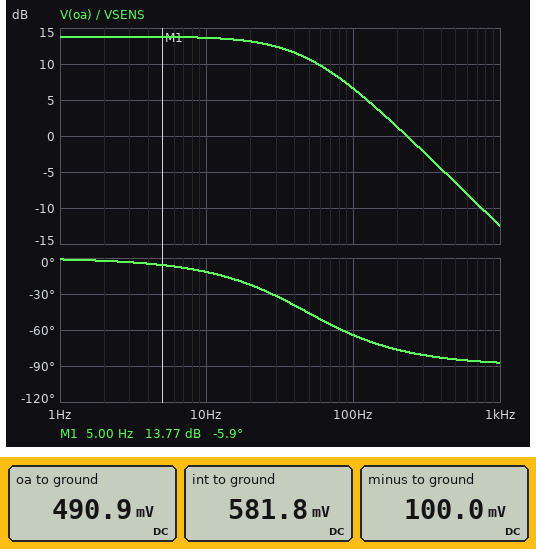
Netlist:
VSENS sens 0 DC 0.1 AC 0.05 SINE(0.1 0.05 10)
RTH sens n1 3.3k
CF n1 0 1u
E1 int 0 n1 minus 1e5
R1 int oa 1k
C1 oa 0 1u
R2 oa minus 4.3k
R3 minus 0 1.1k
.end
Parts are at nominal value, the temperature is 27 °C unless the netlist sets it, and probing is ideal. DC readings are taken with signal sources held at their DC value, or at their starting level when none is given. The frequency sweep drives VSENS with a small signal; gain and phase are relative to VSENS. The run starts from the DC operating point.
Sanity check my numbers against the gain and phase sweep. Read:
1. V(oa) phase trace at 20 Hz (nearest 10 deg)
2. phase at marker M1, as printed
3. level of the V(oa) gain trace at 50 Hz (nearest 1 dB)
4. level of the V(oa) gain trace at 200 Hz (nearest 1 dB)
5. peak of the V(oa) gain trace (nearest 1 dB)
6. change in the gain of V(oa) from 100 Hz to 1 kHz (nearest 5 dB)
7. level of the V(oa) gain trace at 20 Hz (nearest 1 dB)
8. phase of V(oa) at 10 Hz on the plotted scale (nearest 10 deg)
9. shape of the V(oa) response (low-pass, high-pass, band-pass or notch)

-20 deg
-5.9 deg
11 dB
1 dB
14 dB
-20 dB
13 dB
-10 deg
low-pass
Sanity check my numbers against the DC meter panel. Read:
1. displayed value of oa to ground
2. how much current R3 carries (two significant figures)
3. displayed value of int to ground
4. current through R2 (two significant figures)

490.9 mV
91 µA
581.8 mV
91 µA
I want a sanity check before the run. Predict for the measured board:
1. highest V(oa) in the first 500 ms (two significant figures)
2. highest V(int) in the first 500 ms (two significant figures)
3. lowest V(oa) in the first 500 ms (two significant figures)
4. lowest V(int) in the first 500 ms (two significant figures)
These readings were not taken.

730 mV
870 mV
250 mV
300 mV
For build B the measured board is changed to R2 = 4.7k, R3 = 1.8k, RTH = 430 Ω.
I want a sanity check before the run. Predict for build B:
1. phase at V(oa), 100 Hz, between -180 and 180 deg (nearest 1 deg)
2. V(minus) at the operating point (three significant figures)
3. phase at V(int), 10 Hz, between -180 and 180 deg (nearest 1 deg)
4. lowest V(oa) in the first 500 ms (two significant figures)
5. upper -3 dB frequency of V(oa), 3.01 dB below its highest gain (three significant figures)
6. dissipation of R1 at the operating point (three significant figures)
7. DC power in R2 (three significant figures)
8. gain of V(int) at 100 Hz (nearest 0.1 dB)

-15 deg
100 mV
2 deg
180 mV
370 Hz
3.09 µW
14.5 µW
13.2 dB
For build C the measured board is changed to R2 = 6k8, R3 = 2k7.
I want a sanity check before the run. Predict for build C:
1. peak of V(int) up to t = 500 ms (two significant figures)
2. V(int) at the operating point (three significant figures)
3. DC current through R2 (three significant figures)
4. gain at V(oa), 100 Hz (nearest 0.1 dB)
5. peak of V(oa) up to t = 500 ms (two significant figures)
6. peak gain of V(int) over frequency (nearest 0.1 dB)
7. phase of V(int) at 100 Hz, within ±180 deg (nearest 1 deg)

580 mV
389 mV
37.0 µA
3.7 dB
520 mV
11.8 dB
-35 deg
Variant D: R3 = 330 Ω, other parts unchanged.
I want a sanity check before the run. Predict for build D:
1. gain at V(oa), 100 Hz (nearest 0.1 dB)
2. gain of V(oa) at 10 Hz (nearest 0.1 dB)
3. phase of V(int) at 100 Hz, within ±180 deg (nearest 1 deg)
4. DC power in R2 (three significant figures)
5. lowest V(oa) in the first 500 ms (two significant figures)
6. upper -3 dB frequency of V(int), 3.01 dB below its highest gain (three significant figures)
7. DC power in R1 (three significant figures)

15.7 dB
22.8 dB
-37 deg
395 µW
720 mV
51.5 Hz
91.8 µW
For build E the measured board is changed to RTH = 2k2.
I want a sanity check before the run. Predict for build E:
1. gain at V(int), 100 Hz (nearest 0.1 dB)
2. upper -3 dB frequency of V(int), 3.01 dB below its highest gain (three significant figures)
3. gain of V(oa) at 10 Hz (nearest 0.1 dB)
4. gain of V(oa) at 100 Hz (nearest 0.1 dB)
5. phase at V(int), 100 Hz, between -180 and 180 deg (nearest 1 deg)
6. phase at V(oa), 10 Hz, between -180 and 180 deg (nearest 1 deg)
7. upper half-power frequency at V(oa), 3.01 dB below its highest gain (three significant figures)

11.7 dB
86.1 Hz
13.7 dB
9.2 dB
-26 deg
-8 deg
72.3 Hz
